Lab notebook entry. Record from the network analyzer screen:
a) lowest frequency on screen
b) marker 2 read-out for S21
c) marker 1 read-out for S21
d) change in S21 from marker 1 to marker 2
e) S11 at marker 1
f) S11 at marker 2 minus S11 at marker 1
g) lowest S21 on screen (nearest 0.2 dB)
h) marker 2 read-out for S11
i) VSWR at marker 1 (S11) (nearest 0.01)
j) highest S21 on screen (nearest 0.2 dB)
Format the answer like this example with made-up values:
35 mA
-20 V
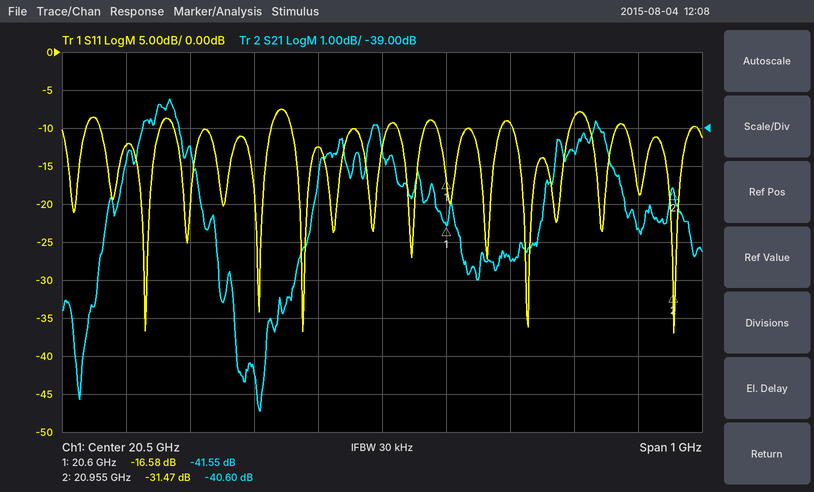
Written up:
20 GHz
-40.60 dB
-41.55 dB
0.95 dB
-16.58 dB
-14.89 dB
-46.4 dB
-31.47 dB
1.35
-38.2 dB
